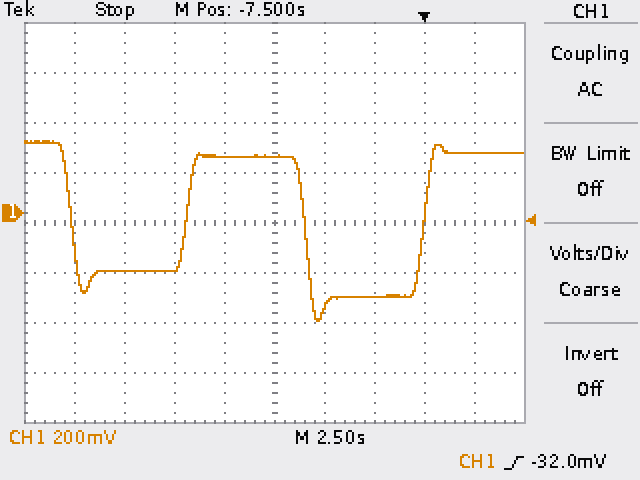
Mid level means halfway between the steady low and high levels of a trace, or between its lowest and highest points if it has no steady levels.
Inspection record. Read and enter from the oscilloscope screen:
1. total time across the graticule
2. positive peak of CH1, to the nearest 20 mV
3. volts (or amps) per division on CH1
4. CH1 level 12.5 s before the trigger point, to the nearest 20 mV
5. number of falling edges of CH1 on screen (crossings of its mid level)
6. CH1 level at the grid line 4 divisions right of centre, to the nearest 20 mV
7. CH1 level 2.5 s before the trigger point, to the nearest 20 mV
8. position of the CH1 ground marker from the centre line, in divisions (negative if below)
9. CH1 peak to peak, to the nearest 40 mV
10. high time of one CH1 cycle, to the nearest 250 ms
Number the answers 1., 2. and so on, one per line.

1. 25 s
2. 280 mV
3. 200 mV
4. -220 mV
5. 2
6. 240 mV
7. -340 mV
8. +0.2 div
9. 720 mV
10. 6.00 s
